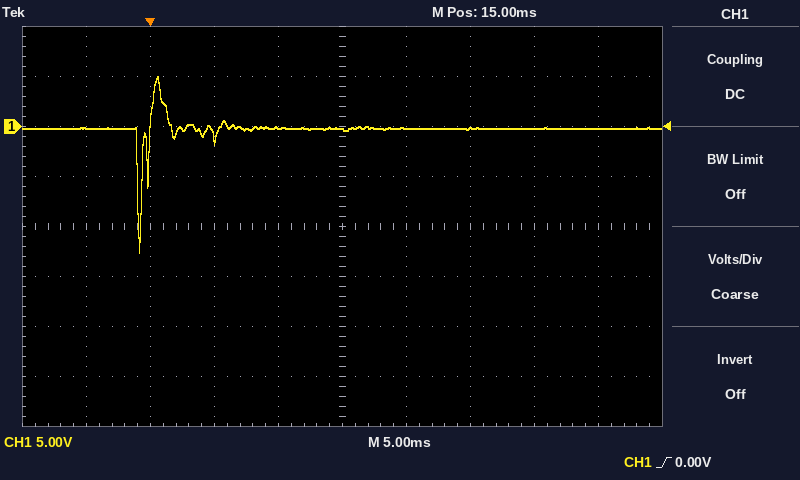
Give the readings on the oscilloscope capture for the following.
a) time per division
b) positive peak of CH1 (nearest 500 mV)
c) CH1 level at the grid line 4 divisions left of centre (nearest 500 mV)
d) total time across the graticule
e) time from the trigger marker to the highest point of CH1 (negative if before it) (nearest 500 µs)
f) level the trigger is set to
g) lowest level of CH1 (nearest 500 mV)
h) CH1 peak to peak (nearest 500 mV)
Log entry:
5 ms
5.0 V
0.0 V
50 ms
+500 µs
0.00 V
-12.5 V
17.5 V
